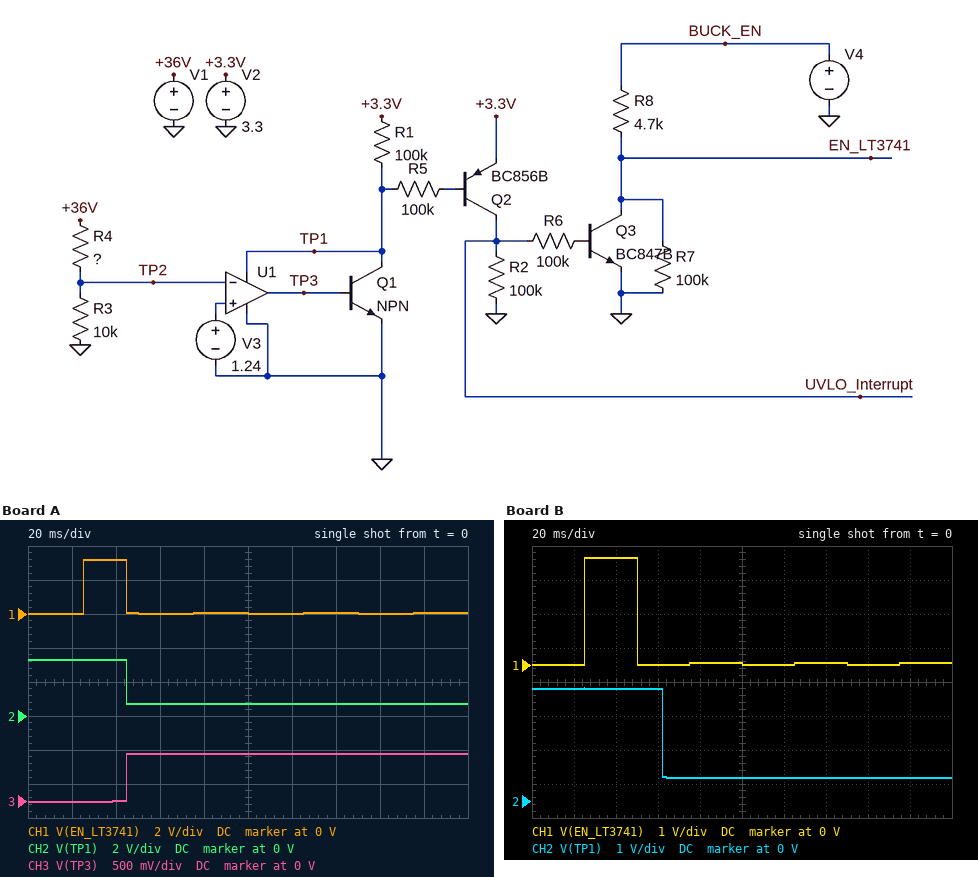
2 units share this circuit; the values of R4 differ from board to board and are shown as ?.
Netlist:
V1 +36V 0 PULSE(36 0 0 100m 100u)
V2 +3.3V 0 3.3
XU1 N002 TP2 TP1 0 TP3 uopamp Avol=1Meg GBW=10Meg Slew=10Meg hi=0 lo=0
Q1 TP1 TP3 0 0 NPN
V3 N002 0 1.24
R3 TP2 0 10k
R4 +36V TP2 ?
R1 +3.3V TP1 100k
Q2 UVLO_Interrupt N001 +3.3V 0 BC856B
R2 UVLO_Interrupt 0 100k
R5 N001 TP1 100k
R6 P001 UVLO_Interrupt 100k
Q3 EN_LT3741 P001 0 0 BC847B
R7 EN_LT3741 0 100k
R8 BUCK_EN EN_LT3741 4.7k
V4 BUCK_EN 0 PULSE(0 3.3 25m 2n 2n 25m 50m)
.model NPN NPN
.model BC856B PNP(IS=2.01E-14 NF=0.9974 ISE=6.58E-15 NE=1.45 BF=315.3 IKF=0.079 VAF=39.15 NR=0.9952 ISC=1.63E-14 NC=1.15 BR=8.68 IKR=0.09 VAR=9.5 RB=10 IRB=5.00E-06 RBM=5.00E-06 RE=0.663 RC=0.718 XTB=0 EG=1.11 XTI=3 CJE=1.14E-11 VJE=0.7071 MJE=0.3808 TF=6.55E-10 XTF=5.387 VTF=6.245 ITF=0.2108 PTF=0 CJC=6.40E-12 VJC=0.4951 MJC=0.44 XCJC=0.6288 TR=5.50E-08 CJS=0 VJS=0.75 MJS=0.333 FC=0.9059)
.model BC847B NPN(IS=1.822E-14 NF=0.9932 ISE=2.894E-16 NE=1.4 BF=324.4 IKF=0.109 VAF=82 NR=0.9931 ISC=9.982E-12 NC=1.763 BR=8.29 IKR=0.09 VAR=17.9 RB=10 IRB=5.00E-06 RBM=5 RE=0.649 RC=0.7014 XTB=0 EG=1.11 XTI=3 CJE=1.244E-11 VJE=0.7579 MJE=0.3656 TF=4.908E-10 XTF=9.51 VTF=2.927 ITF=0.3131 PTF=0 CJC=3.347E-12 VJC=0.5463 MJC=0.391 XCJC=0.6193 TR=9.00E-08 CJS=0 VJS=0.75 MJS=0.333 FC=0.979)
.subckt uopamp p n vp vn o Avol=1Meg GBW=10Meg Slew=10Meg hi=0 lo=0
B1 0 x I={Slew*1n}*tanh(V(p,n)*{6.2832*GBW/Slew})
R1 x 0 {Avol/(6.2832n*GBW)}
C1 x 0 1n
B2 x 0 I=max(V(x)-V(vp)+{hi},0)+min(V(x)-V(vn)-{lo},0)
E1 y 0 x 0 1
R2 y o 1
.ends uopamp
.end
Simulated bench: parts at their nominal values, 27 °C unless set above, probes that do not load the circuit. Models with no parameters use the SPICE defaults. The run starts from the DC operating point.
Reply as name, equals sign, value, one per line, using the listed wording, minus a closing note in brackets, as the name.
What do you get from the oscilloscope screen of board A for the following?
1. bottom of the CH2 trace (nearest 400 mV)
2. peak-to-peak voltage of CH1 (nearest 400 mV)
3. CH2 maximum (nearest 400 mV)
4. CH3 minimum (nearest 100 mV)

bottom of the CH2 trace = 800 mV
peak-to-peak voltage of CH1 = 3.2 V
CH2 maximum = 3.2 V
CH3 minimum = 0 V
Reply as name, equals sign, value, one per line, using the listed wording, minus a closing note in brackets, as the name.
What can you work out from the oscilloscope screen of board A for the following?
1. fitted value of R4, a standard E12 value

fitted value of R4, a standard E12 value = 150 kΩ
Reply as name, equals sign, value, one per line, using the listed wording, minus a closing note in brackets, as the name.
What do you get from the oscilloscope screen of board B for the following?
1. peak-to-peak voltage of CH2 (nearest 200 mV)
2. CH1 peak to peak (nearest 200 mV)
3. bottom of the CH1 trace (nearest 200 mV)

peak-to-peak voltage of CH2 = 2.6 V
CH1 peak to peak = 3.2 V
bottom of the CH1 trace = 0 V
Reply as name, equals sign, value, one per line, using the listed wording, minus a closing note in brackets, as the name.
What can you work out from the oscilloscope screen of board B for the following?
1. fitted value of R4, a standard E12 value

fitted value of R4, a standard E12 value = 100 kΩ
